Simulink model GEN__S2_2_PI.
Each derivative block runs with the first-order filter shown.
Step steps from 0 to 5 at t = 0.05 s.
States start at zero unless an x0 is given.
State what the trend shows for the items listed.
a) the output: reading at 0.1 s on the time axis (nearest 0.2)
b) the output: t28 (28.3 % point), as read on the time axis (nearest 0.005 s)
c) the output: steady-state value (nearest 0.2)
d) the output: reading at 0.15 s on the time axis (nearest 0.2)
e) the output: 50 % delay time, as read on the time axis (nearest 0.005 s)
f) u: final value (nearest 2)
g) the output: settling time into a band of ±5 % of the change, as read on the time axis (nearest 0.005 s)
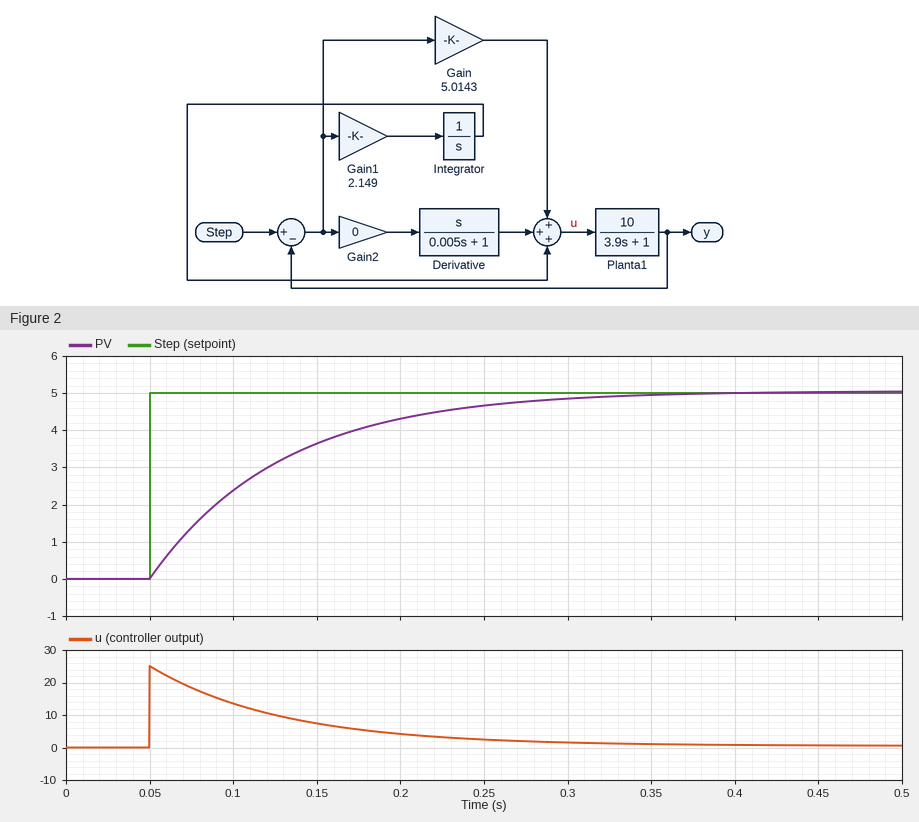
2.4
0.075 s
5.0
3.6
0.105 s
0
0.275 s
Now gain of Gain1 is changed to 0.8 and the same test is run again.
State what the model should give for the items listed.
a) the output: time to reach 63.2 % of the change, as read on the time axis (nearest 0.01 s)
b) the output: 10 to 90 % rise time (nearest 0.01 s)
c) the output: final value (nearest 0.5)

0.13 s
0.17 s
5.0
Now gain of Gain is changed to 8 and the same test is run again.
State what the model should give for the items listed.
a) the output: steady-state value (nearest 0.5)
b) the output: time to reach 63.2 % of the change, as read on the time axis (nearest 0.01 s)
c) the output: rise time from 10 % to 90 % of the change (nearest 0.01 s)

5.0
0.10 s
0.11 s
